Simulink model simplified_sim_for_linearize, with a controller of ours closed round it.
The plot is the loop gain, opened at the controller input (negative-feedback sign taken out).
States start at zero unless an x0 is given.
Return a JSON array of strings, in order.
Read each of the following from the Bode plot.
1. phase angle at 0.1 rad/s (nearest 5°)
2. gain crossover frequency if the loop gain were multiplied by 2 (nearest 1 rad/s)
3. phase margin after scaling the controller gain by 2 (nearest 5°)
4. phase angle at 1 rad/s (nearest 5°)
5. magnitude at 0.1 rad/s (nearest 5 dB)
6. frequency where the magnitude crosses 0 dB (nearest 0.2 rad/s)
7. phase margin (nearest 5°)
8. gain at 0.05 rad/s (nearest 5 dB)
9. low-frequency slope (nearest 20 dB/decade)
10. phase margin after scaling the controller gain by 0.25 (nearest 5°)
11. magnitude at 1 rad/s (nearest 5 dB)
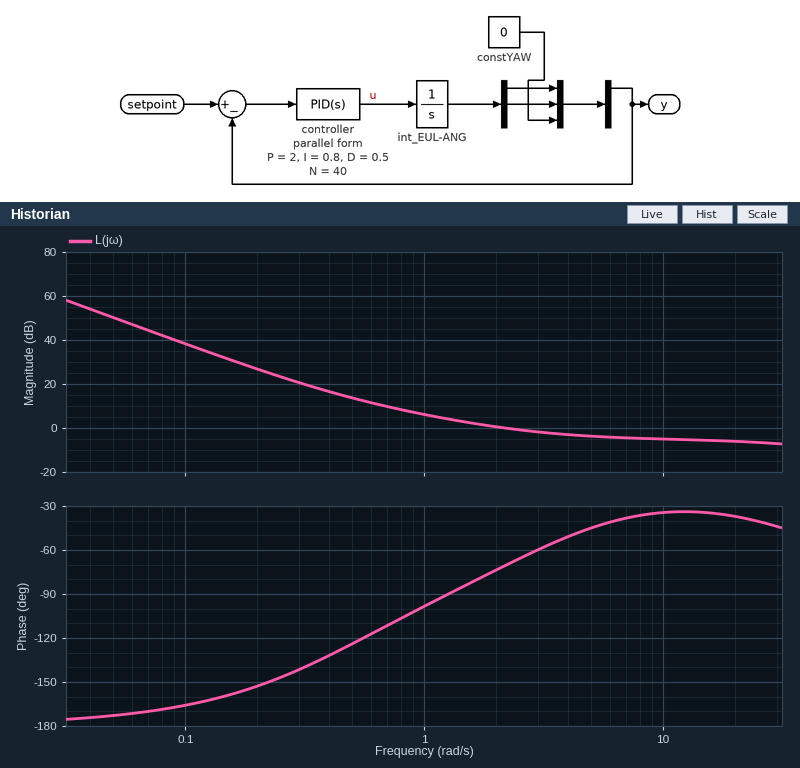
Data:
["-165°", "20 rad/s", "145°", "-100°", "40 dB", "2.2 rad/s", "110°", "50 dB", "-40 dB/decade", "60°", "5 dB"]
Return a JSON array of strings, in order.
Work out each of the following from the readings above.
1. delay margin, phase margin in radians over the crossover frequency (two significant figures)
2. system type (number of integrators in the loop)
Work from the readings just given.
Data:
["0.87 s", "2"]
